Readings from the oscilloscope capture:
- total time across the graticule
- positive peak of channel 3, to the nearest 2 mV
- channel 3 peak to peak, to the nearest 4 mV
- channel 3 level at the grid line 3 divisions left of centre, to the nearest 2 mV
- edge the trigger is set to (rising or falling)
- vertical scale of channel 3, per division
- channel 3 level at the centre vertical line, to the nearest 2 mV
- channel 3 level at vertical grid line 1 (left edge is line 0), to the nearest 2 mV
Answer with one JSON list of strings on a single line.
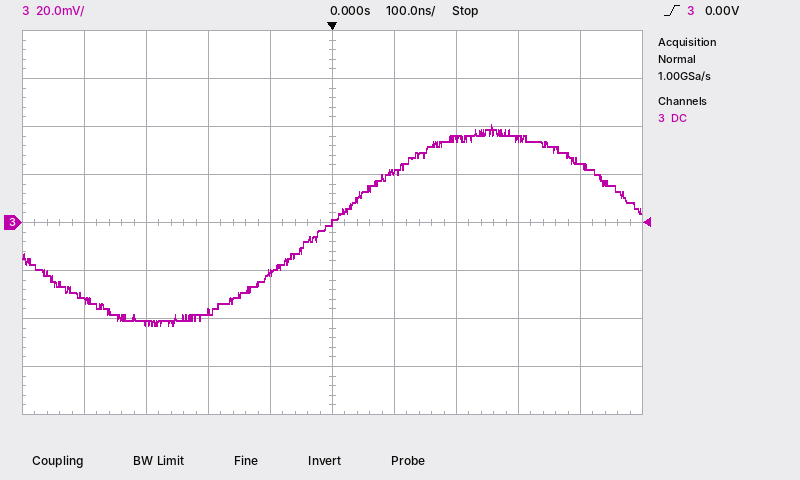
["1 µs", "40 mV", "84 mV", "-42 mV", "rising", "20 mV", "0 mV", "-32 mV"]
